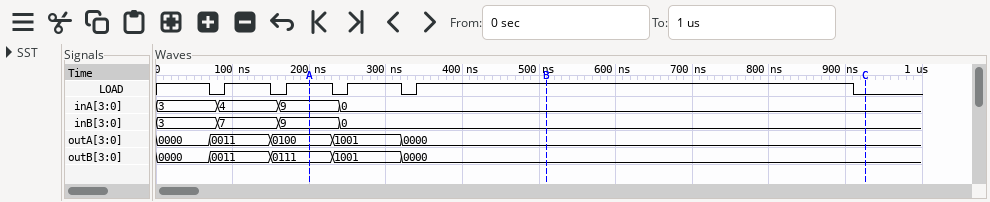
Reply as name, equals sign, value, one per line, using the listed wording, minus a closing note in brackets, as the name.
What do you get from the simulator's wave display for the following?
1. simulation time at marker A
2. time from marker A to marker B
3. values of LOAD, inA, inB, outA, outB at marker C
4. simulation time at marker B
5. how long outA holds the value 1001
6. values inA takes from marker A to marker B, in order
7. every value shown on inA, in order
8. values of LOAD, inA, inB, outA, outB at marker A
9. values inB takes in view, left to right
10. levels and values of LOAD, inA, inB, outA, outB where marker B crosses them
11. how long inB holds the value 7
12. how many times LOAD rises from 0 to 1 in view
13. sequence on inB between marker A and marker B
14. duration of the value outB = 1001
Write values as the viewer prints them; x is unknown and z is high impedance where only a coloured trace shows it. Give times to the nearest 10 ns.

simulation time at marker A = 200 ns
time from marker A to marker B = 310 ns
values of LOAD, inA, inB, outA, outB at marker C = LOAD=0, inA=0, inB=0, outA=0000, outB=0000
simulation time at marker B = 510 ns
how long outA holds the value 1001 = 90 ns
values inA takes from marker A to marker B, in order = 9, 0
every value shown on inA, in order = 3, 4, 9, 0
values of LOAD, inA, inB, outA, outB at marker A = LOAD=1, inA=9, inB=9, outA=0100, outB=0111
values inB takes in view, left to right = 3, 7, 9, 0
levels and values of LOAD, inA, inB, outA, outB where marker B crosses them = LOAD=1, inA=0, inB=0, outA=0000, outB=0000
how long inB holds the value 7 = 80 ns
how many times LOAD rises from 0 to 1 in view = 4
sequence on inB between marker A and marker B = 9, 0
duration of the value outB = 1001 = 90 ns
